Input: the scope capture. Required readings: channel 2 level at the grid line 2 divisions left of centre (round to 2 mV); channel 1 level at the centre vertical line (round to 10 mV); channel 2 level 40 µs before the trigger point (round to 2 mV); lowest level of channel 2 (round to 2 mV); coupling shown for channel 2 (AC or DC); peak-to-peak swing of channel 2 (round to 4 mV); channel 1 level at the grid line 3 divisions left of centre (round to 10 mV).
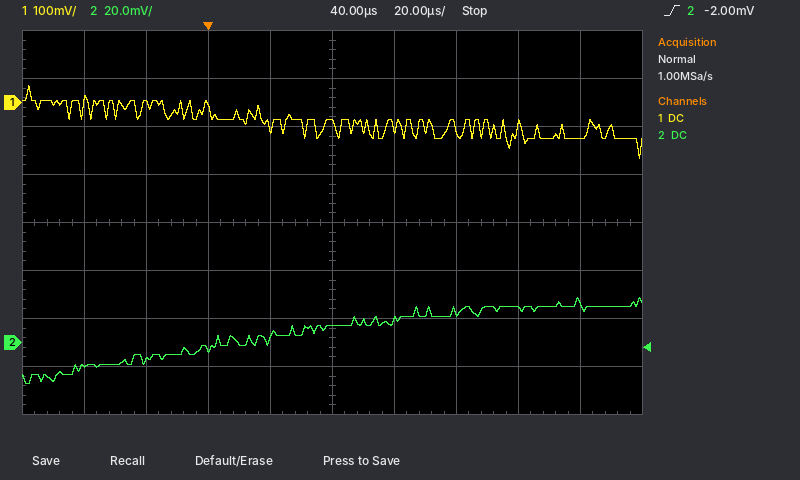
-2 mV
-40 mV
-10 mV
-18 mV
DC
36 mV
0 mV
